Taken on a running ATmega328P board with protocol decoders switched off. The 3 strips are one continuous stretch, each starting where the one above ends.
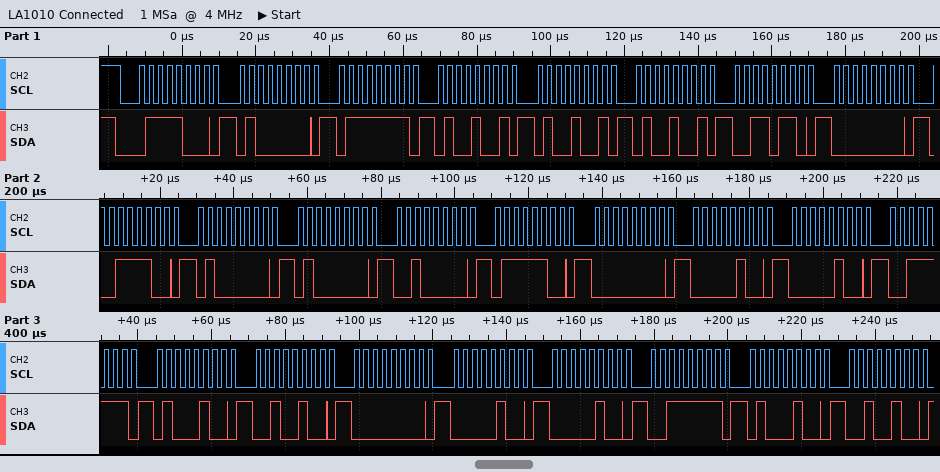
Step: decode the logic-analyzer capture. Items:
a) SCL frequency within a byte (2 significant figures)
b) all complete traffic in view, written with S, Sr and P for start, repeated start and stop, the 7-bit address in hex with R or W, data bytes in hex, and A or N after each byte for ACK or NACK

400 kHz
S 3CW A 40 A 7F A 49 A 49 A 49 A 36 A 00 A 3C A 40 A 40 A 20 A 7C A 00 A 04 A 04 A 3F A 44 A 24 A 00 A 04 A 04 A 3F A 44 A 24 A
